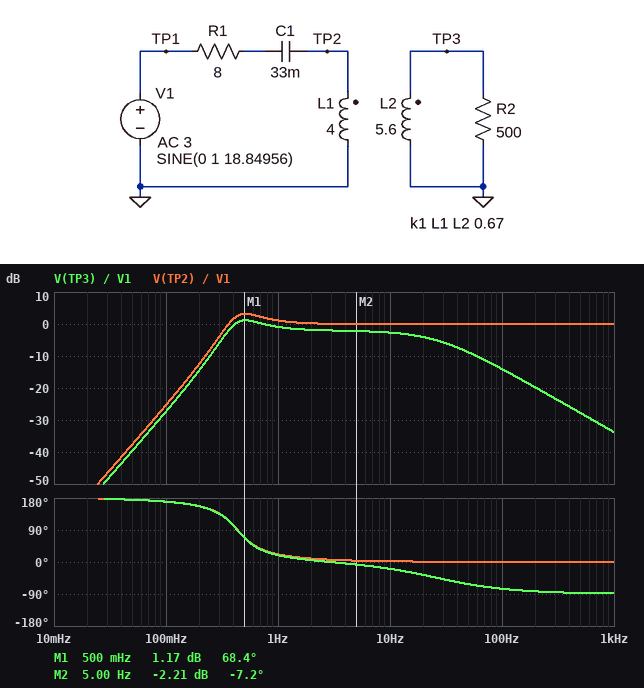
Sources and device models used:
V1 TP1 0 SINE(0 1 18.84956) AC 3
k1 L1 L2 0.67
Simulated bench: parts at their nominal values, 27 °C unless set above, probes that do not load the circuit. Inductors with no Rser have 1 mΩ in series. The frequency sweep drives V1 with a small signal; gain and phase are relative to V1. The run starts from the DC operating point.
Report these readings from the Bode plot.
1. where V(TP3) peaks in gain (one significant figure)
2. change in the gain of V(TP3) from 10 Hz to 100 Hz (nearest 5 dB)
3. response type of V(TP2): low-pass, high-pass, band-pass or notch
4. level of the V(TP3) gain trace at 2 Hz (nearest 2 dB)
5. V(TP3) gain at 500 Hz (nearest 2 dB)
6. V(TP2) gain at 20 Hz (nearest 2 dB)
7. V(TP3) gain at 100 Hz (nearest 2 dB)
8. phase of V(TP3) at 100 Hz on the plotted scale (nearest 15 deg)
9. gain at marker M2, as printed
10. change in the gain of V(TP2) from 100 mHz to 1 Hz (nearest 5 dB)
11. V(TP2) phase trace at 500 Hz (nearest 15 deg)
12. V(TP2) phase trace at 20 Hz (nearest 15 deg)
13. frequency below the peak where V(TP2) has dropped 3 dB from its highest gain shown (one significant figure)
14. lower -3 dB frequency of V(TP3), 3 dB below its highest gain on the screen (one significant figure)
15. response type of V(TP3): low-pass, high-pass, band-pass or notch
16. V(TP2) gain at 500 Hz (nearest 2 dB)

500 mHz
-10 dB
high-pass
-2 dB
-28 dB
0 dB
-14 dB
-75 deg
-2.21 dB
25 dB
0 deg
0 deg
400 mHz
400 mHz
band-pass
0 dB
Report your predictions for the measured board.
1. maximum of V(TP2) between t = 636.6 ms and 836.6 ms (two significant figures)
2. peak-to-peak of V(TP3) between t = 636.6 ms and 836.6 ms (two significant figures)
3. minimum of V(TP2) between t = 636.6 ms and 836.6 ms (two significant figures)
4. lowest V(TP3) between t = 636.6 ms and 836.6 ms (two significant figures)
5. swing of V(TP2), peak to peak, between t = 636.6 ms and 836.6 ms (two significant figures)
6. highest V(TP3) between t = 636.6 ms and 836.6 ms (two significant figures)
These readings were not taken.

990 mV
1.3 V
-1.0 V
-640 mV
2.0 V
630 mV
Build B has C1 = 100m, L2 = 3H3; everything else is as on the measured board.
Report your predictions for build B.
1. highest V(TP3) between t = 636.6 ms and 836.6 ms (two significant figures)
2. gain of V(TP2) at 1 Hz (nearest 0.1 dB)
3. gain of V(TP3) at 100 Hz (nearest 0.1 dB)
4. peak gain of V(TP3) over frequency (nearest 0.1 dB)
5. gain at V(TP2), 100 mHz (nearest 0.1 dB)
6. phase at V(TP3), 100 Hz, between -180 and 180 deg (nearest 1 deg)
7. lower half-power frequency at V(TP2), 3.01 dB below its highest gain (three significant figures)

550 mV
0 dB
-12.3 dB
-4.2 dB
-15.9 dB
-66 deg
231 mHz
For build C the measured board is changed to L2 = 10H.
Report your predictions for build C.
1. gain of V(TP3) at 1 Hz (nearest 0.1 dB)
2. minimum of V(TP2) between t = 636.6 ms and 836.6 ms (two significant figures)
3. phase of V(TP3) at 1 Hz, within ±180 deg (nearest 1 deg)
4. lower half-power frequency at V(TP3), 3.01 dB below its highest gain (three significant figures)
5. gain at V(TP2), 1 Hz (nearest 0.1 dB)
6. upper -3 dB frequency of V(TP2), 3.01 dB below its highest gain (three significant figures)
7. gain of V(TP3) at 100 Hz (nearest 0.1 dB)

1.5 dB
-1.0 V
18 deg
365 mHz
1.0 dB
2.52 Hz
-16.4 dB
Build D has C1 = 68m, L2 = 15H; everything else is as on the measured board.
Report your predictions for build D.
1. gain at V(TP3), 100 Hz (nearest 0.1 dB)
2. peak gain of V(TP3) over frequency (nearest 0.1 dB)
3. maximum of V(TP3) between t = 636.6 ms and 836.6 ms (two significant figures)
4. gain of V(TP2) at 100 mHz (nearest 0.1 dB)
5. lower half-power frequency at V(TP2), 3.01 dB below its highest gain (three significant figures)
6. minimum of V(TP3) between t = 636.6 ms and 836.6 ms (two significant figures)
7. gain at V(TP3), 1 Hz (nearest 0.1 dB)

-18.1 dB
3.0 dB
580 mV
-19.0 dB
260 mHz
-600 mV
2.3 dB
